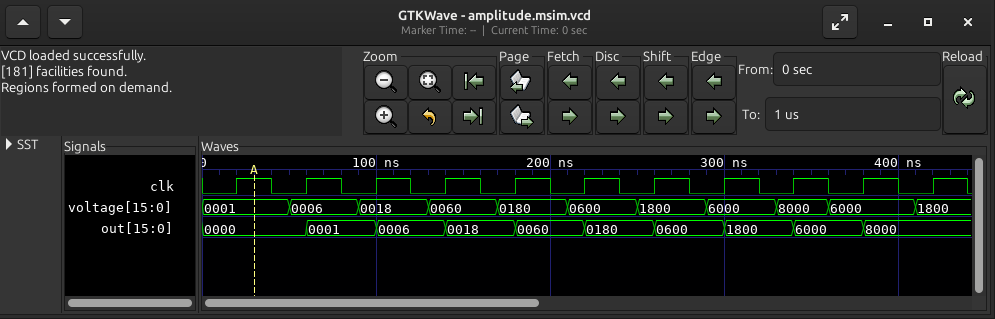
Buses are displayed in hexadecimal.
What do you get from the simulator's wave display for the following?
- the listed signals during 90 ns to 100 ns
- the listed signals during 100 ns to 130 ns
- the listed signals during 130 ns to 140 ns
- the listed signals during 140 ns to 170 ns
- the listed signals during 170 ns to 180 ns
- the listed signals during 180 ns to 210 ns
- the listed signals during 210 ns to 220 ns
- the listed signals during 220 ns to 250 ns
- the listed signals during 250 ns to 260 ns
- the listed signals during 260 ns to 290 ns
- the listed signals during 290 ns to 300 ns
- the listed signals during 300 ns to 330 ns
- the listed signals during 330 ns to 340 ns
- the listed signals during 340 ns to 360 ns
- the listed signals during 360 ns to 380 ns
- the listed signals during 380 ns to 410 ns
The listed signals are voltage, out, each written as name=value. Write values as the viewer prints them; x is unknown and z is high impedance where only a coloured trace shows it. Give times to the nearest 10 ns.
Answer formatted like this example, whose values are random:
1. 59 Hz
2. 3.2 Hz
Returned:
1. voltage=0018, out=0001
2. voltage=0018, out=0006
3. voltage=0060, out=0006
4. voltage=0060, out=0018
5. voltage=0180, out=0018
6. voltage=0180, out=0060
7. voltage=0600, out=0060
8. voltage=0600, out=0180
9. voltage=1800, out=0180
10. voltage=1800, out=0600
11. voltage=6000, out=0600
12. voltage=6000, out=1800
13. voltage=8000, out=1800
14. voltage=8000, out=6000
15. voltage=6000, out=6000
16. voltage=6000, out=8000
